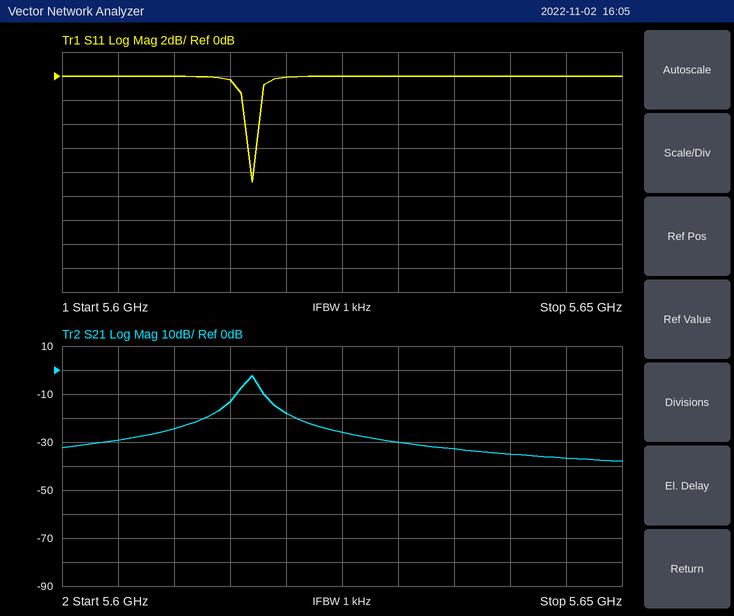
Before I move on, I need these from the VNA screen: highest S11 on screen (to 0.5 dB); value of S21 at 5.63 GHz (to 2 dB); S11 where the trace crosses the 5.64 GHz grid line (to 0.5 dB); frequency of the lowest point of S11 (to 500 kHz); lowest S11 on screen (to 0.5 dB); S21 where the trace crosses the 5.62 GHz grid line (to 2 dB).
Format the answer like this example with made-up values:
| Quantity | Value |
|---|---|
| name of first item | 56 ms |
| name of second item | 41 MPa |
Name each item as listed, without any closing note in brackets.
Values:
| Quantity | Value |
|---|---|
| highest S11 on screen | 0.0 dB |
| value of S21 at 5.63 GHz | -30 dB |
| S11 where the trace crosses the 5.64 GHz grid line | 0.0 dB |
| frequency of the lowest point of S11 | 5.6170 GHz |
| lowest S11 on screen | -9.0 dB |
| S21 where the trace crosses the 5.62 GHz grid line | -18 dB |
